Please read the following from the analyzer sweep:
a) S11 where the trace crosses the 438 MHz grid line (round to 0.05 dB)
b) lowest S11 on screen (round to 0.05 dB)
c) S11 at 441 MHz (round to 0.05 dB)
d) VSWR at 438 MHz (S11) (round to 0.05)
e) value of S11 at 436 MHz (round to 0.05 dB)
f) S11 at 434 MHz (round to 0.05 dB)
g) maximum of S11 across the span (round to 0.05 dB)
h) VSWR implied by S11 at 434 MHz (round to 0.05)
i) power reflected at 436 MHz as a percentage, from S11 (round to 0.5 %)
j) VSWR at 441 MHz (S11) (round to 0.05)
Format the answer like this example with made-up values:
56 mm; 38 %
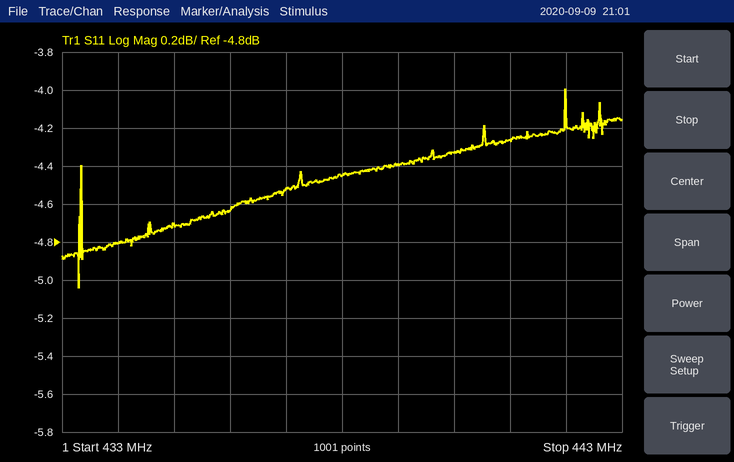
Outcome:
-4.45 dB; -5.05 dB; -4.25 dB; 4.00; -4.65 dB; -4.80 dB; -4.00 dB; 3.70; 34.5 %; 4.15
